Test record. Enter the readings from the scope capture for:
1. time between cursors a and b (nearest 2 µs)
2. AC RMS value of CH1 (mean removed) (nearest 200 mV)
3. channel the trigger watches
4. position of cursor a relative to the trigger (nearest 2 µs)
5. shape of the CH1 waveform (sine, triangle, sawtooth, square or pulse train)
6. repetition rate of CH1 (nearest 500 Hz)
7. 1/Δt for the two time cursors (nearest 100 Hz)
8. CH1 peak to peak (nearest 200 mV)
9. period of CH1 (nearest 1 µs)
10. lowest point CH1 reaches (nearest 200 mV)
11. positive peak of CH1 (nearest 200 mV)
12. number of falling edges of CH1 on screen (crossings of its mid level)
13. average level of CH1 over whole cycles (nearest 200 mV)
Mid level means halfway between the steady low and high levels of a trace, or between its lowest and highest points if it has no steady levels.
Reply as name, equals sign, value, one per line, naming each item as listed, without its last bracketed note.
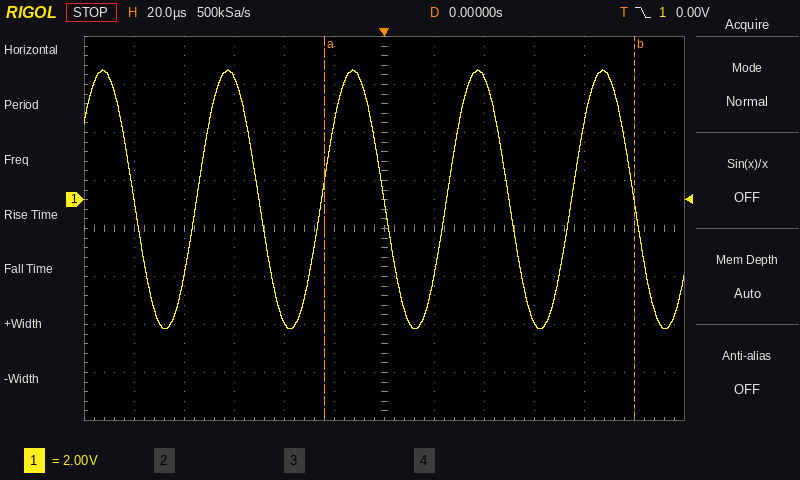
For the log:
time between cursors a and b = 124 µs
AC RMS value of CH1 (mean removed) = 3.8 V
channel the trigger watches = CH1
position of cursor a relative to the trigger = -24 µs
shape of the CH1 waveform = sine
repetition rate of CH1 = 20.0 kHz
1/Δt for the two time cursors = 8.1 kHz
CH1 peak to peak = 10.8 V
period of CH1 = 50 µs
lowest point CH1 reaches = -5.4 V
positive peak of CH1 = 5.4 V
number of falling edges of CH1 on screen = 5
average level of CH1 over whole cycles = 0.0 V
